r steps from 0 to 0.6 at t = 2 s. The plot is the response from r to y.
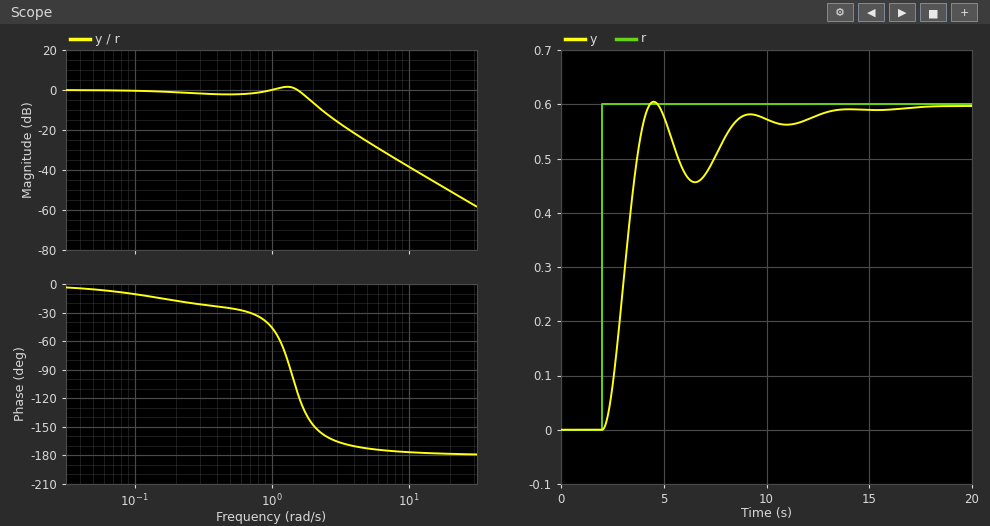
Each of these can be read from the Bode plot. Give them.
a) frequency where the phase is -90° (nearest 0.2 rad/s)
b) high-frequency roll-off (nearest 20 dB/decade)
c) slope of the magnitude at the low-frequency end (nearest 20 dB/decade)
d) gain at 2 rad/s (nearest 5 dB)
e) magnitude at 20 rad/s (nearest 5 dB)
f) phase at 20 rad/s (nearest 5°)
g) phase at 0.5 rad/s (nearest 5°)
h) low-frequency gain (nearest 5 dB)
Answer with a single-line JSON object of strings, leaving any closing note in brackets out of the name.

{"frequency where the phase is -90°": "1.4 rad/s", "high-frequency roll-off": "-40 dB/decade", "slope of the magnitude at the low-frequency end": "0 dB/decade", "gain at 2 rad/s": "-5 dB", "magnitude at 20 rad/s": "-50 dB", "phase at 20 rad/s": "-180°", "phase at 0.5 rad/s": "-25°", "low-frequency gain": "0 dB"}
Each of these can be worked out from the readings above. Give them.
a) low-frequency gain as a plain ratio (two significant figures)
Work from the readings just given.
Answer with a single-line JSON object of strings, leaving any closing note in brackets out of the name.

{"low-frequency gain as a plain ratio": "1.0"}
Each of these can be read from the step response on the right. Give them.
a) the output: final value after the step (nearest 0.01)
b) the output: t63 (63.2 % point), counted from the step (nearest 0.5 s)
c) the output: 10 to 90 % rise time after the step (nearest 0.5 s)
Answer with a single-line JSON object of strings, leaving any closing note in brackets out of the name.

{"the output: final value after the step": "0.60", "the output: t63 (63.2 % point), counted from the step": "1.5 s", "the output: 10 to 90 % rise time after the step": "1.5 s"}
